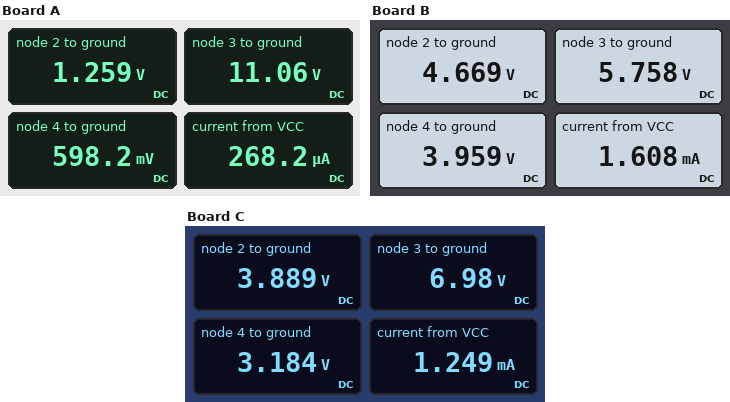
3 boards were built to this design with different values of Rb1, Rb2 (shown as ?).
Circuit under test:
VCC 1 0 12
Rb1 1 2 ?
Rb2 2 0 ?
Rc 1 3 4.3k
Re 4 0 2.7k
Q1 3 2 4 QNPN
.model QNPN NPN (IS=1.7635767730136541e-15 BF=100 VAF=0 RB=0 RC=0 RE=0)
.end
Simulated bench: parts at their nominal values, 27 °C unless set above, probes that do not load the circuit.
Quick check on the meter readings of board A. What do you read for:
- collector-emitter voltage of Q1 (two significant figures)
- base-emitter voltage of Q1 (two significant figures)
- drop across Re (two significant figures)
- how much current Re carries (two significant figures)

10 V
660 mV
600 mV
220 µA
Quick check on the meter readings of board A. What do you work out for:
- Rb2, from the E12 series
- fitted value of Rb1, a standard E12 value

27 kΩ
220 kΩ
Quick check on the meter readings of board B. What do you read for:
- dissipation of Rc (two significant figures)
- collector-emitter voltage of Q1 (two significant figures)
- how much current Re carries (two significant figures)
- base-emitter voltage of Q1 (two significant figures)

9.1 mW
1.8 V
1.5 mA
710 mV
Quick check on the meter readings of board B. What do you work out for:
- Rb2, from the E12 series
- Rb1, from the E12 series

33 kΩ
47 kΩ
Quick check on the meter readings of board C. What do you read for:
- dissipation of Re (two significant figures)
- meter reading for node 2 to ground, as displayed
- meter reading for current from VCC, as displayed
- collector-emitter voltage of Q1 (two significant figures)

3.8 mW
3.889 V
1.249 mA
3.8 V
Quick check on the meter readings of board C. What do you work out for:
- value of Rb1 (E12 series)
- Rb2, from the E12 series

100 kΩ
56 kΩ
